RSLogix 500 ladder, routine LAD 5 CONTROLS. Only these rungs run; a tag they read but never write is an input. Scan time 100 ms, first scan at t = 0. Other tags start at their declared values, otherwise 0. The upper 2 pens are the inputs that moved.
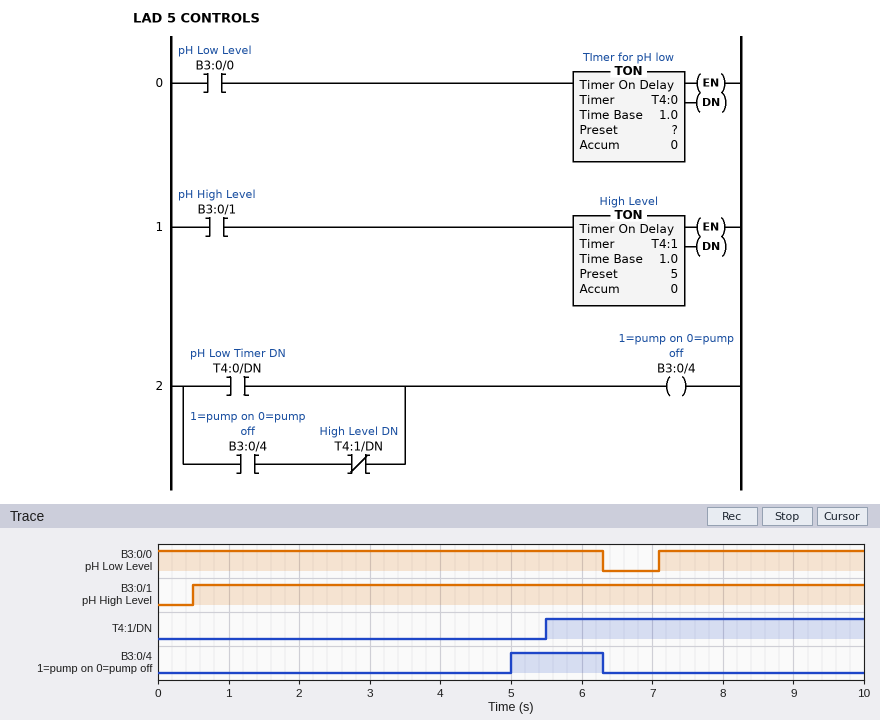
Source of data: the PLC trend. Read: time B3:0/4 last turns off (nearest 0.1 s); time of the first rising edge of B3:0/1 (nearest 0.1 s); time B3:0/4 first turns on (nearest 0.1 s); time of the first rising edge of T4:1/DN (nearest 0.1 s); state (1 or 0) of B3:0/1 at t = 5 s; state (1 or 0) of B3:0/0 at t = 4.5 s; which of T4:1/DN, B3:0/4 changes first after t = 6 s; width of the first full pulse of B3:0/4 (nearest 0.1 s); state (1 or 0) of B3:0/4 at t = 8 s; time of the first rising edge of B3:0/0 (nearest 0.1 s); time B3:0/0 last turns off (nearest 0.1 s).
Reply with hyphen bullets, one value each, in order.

- 6.3 s
- 0.5 s
- 5.0 s
- 5.5 s
- 1
- 1
- B3:0/4
- 1.3 s
- 0
- 7.1 s
- 6.3 s
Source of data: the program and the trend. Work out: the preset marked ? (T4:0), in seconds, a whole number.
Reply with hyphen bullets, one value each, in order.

- 5 s
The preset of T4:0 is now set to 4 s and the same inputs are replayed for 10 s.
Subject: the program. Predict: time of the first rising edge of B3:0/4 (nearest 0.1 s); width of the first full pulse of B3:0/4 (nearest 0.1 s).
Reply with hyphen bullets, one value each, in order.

- 4.0 s
- 2.3 s
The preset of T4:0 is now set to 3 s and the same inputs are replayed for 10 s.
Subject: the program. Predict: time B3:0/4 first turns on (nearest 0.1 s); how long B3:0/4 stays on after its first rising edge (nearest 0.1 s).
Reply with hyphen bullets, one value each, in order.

- 3.0 s
- 3.3 s
